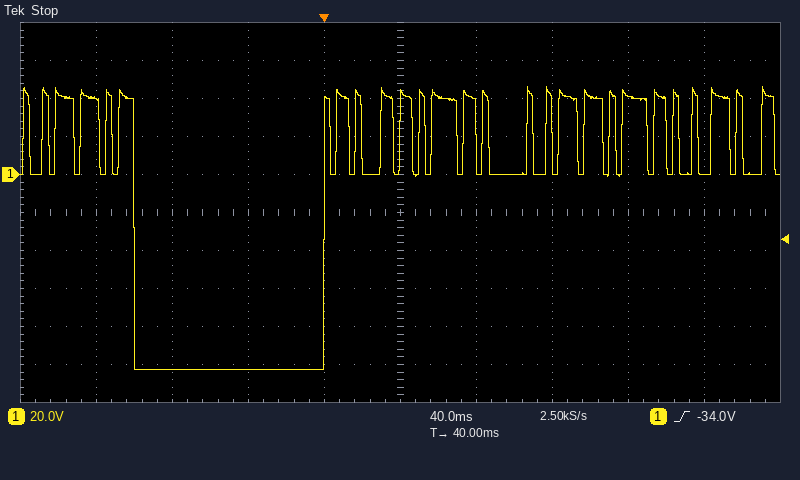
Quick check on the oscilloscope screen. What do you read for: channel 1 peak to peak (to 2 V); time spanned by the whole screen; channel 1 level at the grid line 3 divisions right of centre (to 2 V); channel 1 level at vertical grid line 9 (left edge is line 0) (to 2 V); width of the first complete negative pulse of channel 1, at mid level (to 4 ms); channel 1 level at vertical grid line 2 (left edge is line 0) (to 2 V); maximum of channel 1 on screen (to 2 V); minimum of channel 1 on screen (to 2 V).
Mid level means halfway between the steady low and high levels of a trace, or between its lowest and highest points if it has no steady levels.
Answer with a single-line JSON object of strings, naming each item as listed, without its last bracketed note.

{"channel 1 peak to peak": "148 V", "time spanned by the whole screen": "400 ms", "channel 1 level at the grid line 3 divisions right of centre": "42 V", "channel 1 level at vertical grid line 9 (left edge is line 0)": "0 V", "width of the first complete negative pulse of channel 1, at mid level": "100 ms", "channel 1 level at vertical grid line 2 (left edge is line 0)": "-102 V", "maximum of channel 1 on screen": "46 V", "minimum of channel 1 on screen": "-102 V"}
